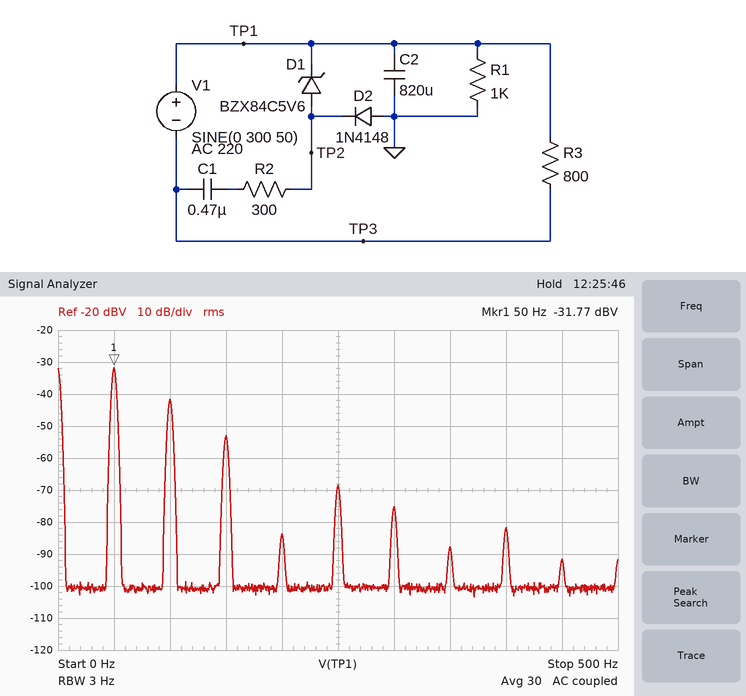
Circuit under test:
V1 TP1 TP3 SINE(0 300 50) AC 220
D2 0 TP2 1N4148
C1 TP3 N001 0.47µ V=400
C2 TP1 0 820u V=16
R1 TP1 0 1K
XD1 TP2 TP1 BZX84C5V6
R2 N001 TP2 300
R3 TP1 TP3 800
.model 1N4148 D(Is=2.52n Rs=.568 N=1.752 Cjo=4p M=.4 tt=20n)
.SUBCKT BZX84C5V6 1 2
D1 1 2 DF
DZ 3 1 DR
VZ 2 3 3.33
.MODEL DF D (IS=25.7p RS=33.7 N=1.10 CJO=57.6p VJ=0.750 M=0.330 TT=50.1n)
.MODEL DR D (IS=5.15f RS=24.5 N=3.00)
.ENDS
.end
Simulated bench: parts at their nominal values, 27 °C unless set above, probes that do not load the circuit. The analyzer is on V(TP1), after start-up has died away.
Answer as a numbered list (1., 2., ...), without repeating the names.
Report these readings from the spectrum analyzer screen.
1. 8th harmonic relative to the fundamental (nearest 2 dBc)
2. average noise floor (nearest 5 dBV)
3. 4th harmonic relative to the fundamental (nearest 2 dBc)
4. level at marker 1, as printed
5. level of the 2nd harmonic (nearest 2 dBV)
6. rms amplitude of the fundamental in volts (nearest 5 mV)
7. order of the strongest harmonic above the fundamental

1. -50 dBc
2. -100 dBV
3. -52 dBc
4. -31.77 dBV
5. -42 dBV
6. 25 mV
7. 2
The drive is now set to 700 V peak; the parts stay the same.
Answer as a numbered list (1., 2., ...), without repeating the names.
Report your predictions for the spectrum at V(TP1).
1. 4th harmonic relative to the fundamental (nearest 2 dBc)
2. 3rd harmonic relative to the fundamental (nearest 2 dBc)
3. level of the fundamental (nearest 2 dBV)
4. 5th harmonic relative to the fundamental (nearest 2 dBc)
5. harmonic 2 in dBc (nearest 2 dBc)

1. -26 dBc
2. -16 dBc
3. -30 dBV
4. -52 dBc
5. -8 dBc
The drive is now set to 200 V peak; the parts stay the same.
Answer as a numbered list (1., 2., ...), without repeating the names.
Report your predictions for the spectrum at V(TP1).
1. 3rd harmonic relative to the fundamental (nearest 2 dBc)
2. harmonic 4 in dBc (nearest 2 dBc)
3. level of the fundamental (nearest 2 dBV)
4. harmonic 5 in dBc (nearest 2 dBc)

1. -26 dBc
2. -36 dBc
3. -32 dBV
4. -38 dBc
